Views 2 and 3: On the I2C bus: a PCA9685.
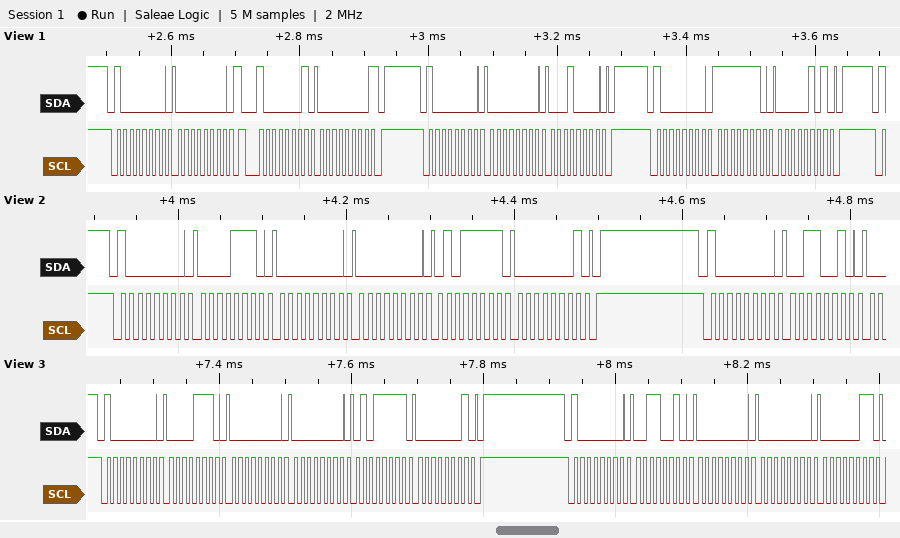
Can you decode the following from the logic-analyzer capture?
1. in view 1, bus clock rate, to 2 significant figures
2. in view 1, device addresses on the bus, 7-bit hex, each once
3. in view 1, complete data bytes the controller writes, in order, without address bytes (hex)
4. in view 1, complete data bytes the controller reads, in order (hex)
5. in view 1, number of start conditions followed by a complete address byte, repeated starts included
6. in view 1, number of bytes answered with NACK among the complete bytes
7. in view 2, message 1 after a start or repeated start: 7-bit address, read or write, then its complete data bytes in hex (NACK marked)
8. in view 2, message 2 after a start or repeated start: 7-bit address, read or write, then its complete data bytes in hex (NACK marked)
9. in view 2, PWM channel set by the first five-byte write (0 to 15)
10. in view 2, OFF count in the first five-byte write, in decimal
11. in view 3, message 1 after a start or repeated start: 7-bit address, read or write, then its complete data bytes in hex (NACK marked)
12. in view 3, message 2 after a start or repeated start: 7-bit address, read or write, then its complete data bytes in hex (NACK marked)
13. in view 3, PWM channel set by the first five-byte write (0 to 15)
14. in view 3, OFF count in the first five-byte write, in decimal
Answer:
100 kHz
0x40
00 00 10 FE 05
00
4
1
0x40 write: 0E 00 00 5F 01
0x40 write: 32
2
351
0x40 write: 0E 00 00 5F 01
0x40 write: 32 00 00 03
2
351
